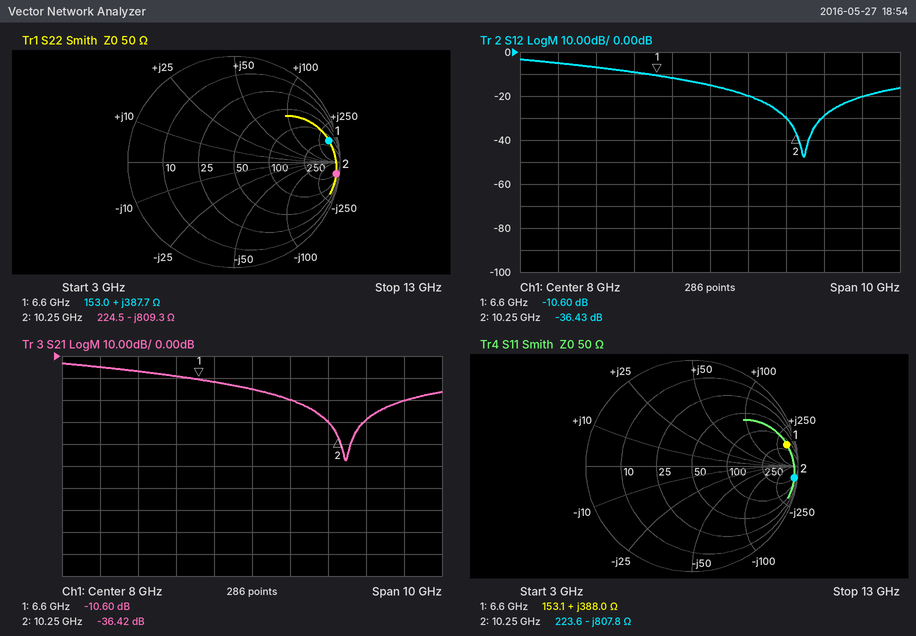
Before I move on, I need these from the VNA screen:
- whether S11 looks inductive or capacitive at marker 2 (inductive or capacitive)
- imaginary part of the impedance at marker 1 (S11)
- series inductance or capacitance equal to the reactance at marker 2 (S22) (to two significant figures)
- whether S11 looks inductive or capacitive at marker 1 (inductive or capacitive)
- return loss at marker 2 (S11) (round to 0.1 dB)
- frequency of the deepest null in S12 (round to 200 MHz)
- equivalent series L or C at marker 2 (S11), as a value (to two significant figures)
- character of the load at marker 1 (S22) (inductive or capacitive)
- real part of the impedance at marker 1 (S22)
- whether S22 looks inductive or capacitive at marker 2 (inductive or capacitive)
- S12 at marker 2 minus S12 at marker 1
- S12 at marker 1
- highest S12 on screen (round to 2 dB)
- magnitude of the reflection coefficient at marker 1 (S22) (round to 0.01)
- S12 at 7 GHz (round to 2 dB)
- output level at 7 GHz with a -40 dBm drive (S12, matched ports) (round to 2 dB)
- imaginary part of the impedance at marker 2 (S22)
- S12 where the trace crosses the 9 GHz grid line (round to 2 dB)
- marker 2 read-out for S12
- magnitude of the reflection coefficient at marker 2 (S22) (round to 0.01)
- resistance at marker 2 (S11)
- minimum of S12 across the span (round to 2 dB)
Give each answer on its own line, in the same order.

capacitive
+388.0 Ω
19 fF
inductive
0.3 dB
10.4 GHz
19 fF
inductive
153.0 Ω
capacitive
-25.83 dB
-10.60 dB
-4 dB
0.92
-12 dB
-52 dBm
-809.3 Ω
-20 dB
-36.43 dB
0.97
223.6 Ω
-48 dB
